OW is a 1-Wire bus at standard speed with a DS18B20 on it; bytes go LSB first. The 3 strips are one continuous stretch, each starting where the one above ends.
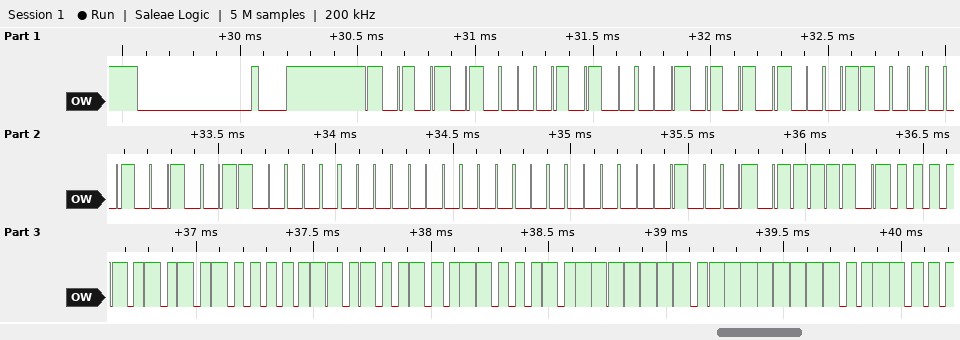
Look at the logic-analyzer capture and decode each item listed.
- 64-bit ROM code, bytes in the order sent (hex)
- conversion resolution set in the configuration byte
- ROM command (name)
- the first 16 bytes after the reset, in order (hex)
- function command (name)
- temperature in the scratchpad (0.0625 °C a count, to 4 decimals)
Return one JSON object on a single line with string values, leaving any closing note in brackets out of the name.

{"64-bit ROM code, bytes in the order sent": "28 54 31 48 06 00 00 88", "conversion resolution set in the configuration byte": "12 bits", "ROM command": "Match ROM", "the first 16 bytes after the reset, in order": "55 28 54 31 48 06 00 00 88 BE 50 05 4B 46 7F FF", "function command": "Read Scratchpad", "temperature in the scratchpad": "85.0000 °C"}
